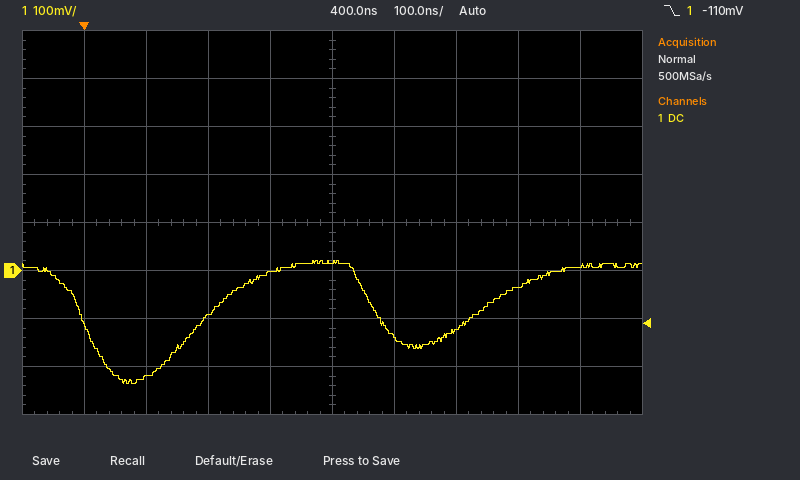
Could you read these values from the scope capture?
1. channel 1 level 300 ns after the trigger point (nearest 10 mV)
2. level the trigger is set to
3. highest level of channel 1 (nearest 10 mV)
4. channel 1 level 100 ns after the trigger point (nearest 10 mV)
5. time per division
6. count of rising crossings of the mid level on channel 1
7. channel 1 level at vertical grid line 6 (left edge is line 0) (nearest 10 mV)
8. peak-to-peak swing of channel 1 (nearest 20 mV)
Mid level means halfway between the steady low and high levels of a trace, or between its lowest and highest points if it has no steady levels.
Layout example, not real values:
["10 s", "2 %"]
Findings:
["0 mV", "-110 mV", "20 mV", "-220 mV", "100 ns", "2", "-140 mV", "260 mV"]
